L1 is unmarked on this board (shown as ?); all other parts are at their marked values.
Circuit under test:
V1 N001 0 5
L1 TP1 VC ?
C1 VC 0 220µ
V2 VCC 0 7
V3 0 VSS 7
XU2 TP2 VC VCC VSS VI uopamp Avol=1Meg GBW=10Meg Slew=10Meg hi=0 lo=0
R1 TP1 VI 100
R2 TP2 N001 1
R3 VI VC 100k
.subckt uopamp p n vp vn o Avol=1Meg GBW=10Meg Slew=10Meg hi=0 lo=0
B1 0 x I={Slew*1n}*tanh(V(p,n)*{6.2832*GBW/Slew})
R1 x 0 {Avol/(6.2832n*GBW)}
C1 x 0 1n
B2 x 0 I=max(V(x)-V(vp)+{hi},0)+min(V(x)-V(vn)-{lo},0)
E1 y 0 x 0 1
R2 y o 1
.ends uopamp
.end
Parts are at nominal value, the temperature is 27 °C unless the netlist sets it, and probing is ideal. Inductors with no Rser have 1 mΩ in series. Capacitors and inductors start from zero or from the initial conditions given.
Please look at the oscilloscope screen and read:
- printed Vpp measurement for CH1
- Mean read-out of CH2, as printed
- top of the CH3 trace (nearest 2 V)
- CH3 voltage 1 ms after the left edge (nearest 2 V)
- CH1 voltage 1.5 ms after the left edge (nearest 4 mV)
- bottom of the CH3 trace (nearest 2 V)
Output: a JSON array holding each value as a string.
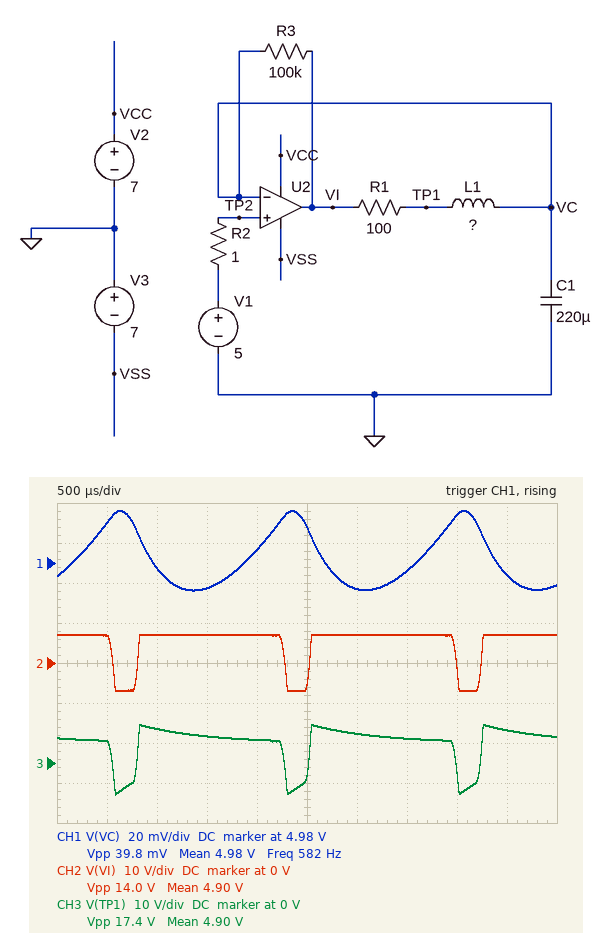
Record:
["39.8 mV", "4.90 V", "10 V", "8 V", "4.968 V", "-8 V"]
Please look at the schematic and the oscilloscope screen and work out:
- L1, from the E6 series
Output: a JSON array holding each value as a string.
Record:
["68 mH"]
